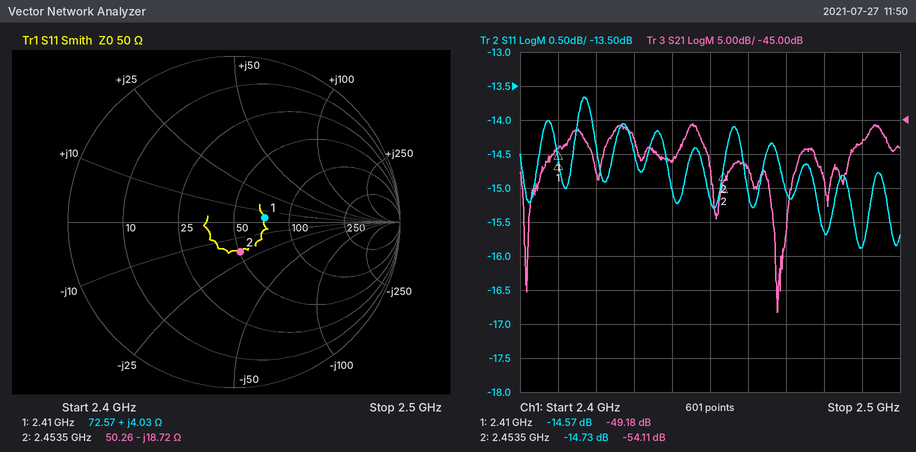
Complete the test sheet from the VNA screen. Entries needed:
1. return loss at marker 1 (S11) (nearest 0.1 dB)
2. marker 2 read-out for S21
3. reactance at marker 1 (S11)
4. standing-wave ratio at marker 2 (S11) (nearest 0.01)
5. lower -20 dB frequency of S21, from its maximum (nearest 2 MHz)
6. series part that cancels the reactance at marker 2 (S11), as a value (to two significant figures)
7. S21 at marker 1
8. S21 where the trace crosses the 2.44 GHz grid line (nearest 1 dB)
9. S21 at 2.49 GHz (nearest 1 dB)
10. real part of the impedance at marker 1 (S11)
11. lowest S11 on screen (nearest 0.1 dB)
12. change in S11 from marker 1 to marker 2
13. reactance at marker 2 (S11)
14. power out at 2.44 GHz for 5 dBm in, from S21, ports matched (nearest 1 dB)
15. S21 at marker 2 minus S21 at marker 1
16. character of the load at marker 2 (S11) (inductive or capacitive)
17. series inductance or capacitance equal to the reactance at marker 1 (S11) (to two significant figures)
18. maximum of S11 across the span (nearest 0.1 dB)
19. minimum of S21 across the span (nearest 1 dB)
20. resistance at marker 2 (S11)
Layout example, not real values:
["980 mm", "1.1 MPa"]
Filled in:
["14.6 dB", "-54.11 dB", "+4.03 Ω", "1.45", "2.402 GHz", "1.2 nH", "-49.18 dB", "-51 dB", "-48 dB", "72.57 Ω", "-15.9 dB", "-0.16 dB", "-18.72 Ω", "-46 dBm", "-4.93 dB", "capacitive", "270 pH", "-13.7 dB", "-73 dB", "50.26 Ω"]
